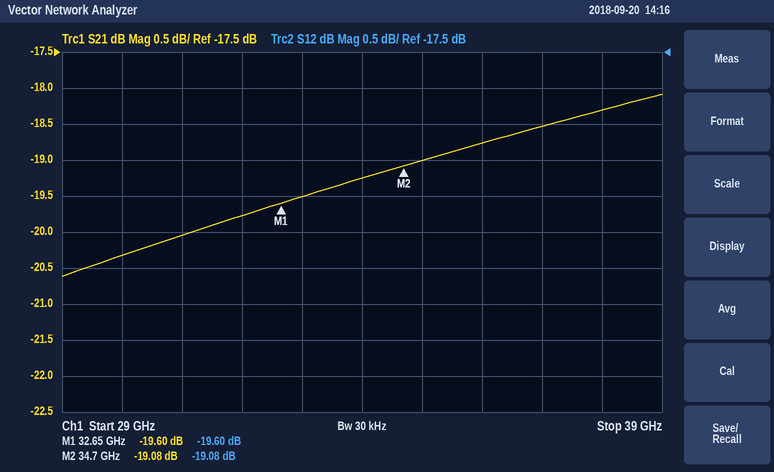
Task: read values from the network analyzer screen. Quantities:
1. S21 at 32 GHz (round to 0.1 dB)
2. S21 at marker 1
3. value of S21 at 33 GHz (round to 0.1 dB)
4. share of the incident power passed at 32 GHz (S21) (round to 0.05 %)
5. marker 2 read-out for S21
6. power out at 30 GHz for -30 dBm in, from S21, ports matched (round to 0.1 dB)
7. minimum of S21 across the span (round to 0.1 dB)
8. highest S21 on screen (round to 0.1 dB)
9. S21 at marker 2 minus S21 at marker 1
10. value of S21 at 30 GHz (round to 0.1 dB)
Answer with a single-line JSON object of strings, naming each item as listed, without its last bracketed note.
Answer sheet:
{"S21 at 32 GHz": "-19.8 dB", "S21 at marker 1": "-19.60 dB", "value of S21 at 33 GHz": "-19.5 dB", "share of the incident power passed at 32 GHz (S21)": "1.05 %", "marker 2 read-out for S21": "-19.08 dB", "power out at 30 GHz for -30 dBm in, from S21, ports matched": "-50.3 dBm", "minimum of S21 across the span": "-20.6 dB", "highest S21 on screen": "-18.1 dB", "S21 at marker 2 minus S21 at marker 1": "0.52 dB", "value of S21 at 30 GHz": "-20.3 dB"}
